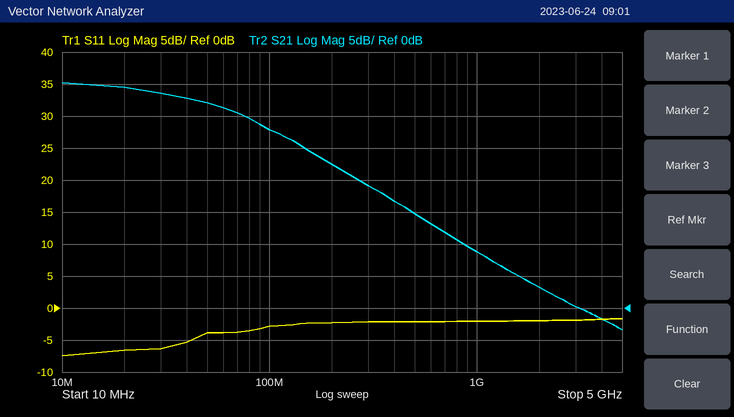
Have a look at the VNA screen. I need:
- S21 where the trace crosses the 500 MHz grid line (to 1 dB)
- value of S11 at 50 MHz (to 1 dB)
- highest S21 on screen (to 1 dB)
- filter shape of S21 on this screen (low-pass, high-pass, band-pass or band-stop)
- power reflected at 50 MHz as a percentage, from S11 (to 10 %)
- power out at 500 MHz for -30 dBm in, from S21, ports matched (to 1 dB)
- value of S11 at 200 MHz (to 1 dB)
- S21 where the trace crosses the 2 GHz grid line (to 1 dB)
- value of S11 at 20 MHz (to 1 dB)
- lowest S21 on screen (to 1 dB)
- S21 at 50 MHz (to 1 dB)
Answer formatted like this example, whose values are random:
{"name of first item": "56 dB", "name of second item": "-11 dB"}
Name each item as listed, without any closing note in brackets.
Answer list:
{"S21 where the trace crosses the 500 MHz grid line": "15 dB", "value of S11 at 50 MHz": "-4 dB", "highest S21 on screen": "35 dB", "filter shape of S21 on this screen": "low-pass", "power reflected at 50 MHz as a percentage, from S11": "40 %", "power out at 500 MHz for -30 dBm in, from S21, ports matched": "-15 dBm", "value of S11 at 200 MHz": "-2 dB", "S21 where the trace crosses the 2 GHz grid line": "3 dB", "value of S11 at 20 MHz": "-7 dB", "lowest S21 on screen": "-3 dB", "S21 at 50 MHz": "32 dB"}
